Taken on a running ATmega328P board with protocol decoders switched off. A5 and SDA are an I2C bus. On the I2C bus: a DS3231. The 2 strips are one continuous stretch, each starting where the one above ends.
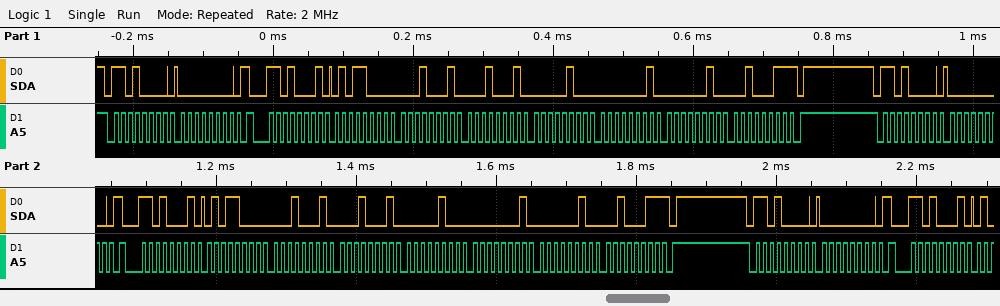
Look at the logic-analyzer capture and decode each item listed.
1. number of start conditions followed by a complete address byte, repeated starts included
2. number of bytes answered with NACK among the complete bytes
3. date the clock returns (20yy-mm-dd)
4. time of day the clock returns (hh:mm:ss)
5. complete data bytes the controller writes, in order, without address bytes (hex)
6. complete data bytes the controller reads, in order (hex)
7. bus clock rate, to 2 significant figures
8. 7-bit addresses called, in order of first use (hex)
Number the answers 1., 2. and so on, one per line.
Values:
1. 6
2. 2
3. 2023-02-01
4. 11:11:58
5. 00 00 00
6. 58 11 11 04 01 02 23 58 11 11 04 01 02 23
7. 100 kHz
8. 0x68
